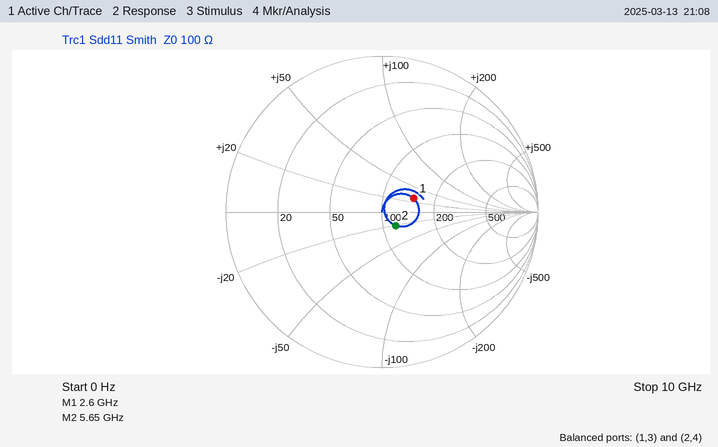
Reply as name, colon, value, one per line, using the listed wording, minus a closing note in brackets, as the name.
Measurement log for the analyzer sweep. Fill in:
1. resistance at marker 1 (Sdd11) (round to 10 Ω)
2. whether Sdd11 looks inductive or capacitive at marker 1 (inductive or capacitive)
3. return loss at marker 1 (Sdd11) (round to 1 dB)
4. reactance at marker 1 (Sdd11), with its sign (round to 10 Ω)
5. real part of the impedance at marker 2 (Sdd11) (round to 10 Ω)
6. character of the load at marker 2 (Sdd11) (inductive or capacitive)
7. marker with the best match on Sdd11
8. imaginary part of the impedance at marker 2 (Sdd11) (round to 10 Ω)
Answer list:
resistance at marker 1 (Sdd11): 150 Ω
whether Sdd11 looks inductive or capacitive at marker 1: inductive
return loss at marker 1 (Sdd11): 13 dB
reactance at marker 1 (Sdd11), with its sign: +30 Ω
real part of the impedance at marker 2 (Sdd11): 120 Ω
character of the load at marker 2 (Sdd11): capacitive
marker with the best match on Sdd11: marker 2
imaginary part of the impedance at marker 2 (Sdd11): -20 Ω
